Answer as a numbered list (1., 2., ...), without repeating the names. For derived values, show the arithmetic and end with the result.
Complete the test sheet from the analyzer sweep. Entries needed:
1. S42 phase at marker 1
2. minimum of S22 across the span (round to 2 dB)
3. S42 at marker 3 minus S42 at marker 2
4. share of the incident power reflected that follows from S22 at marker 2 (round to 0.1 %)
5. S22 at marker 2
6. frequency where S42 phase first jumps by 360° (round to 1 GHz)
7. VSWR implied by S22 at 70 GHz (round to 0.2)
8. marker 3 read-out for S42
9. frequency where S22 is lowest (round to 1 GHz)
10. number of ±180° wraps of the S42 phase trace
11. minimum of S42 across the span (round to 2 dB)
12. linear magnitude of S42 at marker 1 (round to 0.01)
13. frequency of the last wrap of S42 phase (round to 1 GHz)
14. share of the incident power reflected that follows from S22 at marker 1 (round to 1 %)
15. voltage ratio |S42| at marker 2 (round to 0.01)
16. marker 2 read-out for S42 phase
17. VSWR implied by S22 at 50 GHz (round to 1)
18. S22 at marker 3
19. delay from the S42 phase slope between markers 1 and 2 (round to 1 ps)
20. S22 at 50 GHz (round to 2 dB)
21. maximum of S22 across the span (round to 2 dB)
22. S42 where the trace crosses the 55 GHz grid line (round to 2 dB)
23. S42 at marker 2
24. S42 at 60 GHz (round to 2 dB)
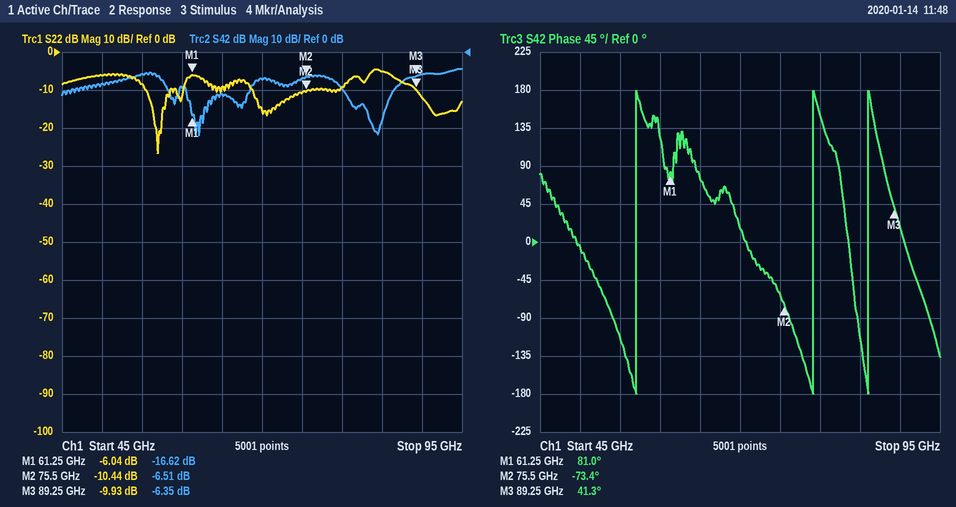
1. 81.0°
2. -26 dB
3. -6.35 − (-6.51) = 0.16 dB
4. 10^(-10.44/10) ≈ 9.0 %
5. -10.44 dB
6. 57 GHz
7. |Γ| = 10^(-16/20) = 0.1585; VSWR = (1 + 0.1585)/(1 − 0.1585) ≈ 1.4
8. -6.35 dB
9. 57 GHz
10. 3
11. -22 dB
12. 10^(-16.62/20) ≈ 0.15
13. 86 GHz
14. 10^(-6.04/10) ≈ 25 %
15. 10^(-6.51/20) ≈ 0.47
16. -73.4°
17. |Γ| = 10^(-6/20) = 0.5012; VSWR = (1 + 0.5012)/(1 − 0.5012) ≈ 3
18. -9.93 dB
19. −(-73.4° − (81°))/(360° × 14.25 GHz) ≈ 30 ps
20. -6 dB
21. -4 dB
22. -6 dB
23. -6.51 dB
24. -10 dB
